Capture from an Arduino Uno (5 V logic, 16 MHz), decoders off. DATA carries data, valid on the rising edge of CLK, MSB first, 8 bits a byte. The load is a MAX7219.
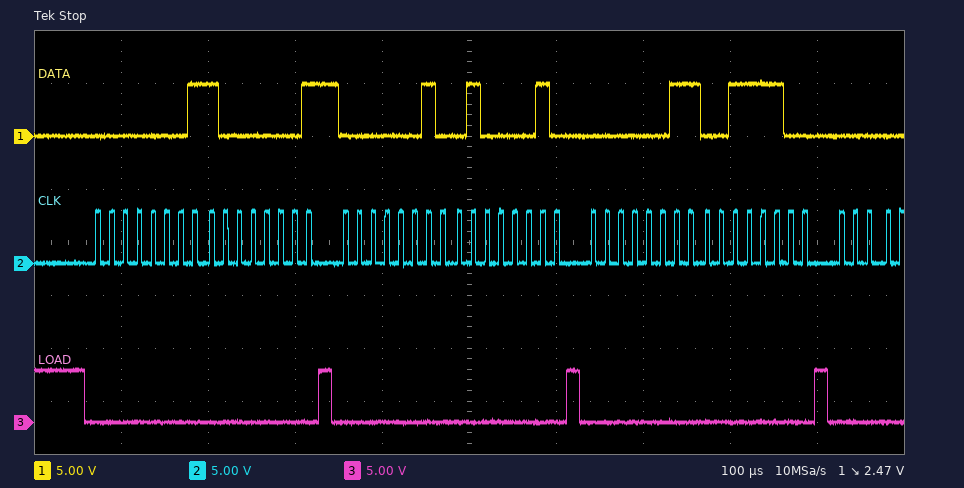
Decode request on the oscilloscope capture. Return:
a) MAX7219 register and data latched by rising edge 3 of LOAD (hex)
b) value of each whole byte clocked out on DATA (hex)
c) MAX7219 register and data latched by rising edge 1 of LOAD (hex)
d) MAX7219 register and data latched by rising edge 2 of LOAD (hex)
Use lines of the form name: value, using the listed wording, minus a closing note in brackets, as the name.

MAX7219 register and data latched by rising edge 3 of LOAD: register 0x3, data 0x3C
value of each whole byte clocked out on DATA: 01 81 02 42 03 3C
MAX7219 register and data latched by rising edge 1 of LOAD: register 0x1, data 0x81
MAX7219 register and data latched by rising edge 2 of LOAD: register 0x2, data 0x42
